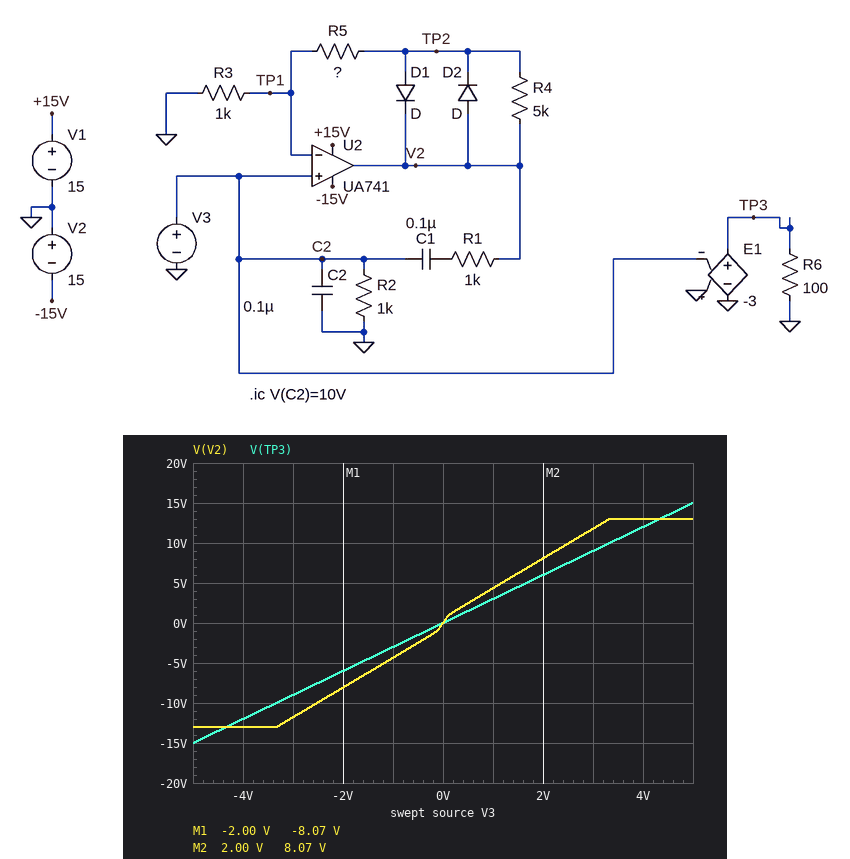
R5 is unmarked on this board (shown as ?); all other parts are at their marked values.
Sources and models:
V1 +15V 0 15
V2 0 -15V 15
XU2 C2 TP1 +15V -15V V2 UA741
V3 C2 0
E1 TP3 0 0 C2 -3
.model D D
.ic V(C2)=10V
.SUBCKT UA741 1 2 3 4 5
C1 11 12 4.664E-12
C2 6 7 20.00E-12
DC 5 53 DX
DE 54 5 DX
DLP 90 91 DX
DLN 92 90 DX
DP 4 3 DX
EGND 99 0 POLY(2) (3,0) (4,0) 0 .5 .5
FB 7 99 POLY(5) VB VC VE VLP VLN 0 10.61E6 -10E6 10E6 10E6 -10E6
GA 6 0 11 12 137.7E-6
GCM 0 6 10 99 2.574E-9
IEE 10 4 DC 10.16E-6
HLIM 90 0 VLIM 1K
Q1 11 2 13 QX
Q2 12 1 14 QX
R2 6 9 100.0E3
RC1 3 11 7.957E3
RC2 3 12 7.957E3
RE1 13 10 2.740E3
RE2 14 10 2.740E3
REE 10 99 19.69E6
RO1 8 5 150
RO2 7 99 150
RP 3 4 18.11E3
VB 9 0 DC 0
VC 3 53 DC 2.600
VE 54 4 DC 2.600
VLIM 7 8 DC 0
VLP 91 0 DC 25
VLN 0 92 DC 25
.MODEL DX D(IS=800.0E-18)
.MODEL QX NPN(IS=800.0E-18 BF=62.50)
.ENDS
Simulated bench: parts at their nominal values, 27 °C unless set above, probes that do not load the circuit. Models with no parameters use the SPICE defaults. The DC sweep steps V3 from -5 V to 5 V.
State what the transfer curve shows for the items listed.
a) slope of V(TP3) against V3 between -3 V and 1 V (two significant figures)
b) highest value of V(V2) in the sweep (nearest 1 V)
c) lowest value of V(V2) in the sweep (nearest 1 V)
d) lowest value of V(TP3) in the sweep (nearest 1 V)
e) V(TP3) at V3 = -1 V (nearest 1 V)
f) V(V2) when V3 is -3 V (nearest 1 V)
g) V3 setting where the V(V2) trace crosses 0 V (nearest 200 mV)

3.0 V/V
13 V
-13 V
-15 V
-3 V
-12 V
0 V
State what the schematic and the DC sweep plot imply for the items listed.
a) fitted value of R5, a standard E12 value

2.7 kΩ
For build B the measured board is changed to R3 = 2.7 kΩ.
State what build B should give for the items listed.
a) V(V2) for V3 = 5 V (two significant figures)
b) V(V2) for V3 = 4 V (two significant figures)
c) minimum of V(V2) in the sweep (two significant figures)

11 V
8.7 V
-11 V
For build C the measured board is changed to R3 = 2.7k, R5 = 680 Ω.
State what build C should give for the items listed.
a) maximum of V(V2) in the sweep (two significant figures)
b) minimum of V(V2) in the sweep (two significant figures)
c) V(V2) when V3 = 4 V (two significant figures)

6.9 V
-6.9 V
5.7 V
